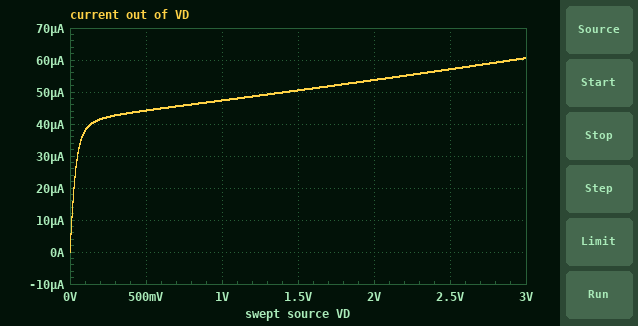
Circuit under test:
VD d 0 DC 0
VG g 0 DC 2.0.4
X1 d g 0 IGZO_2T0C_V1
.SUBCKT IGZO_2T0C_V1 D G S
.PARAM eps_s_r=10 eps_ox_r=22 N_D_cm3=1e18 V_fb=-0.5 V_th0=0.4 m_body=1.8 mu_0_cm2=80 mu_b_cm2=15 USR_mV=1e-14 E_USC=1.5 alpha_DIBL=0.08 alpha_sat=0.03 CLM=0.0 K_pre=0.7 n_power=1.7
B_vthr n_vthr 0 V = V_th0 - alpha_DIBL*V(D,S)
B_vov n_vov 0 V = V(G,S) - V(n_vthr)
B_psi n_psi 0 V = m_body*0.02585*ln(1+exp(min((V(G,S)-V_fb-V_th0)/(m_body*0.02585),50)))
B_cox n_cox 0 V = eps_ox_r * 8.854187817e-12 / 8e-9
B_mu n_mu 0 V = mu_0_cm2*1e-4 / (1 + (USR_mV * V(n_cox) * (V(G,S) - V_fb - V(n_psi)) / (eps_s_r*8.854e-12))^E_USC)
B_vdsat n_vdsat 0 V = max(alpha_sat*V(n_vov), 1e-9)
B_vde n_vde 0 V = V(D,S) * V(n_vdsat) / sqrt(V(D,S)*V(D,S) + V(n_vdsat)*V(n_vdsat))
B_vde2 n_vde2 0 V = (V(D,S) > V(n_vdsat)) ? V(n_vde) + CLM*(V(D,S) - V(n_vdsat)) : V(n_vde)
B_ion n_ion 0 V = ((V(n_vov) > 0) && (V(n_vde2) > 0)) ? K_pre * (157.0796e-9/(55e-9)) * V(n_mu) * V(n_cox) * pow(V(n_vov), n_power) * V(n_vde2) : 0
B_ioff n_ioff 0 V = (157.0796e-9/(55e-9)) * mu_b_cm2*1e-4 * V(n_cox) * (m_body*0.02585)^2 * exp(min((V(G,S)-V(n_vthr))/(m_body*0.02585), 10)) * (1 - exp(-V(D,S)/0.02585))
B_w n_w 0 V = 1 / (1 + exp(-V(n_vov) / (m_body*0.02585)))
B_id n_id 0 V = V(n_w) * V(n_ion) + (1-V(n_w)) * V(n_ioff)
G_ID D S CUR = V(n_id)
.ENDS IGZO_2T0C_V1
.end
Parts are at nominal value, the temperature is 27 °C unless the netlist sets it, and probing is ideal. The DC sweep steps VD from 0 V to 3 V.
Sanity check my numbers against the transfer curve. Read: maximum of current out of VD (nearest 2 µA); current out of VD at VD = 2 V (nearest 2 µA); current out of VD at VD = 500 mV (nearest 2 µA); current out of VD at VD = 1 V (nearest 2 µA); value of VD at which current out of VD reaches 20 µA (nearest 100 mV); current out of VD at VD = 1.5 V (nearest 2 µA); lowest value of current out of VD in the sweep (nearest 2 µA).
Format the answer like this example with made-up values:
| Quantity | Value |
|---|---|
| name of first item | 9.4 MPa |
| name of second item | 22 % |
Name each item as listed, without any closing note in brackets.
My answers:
| Quantity | Value |
|---|---|
| maximum of current out of VD | 60 µA |
| current out of VD at VD = 2 V | 54 µA |
| current out of VD at VD = 500 mV | 44 µA |
| current out of VD at VD = 1 V | 48 µA |
| value of VD at which current out of VD reaches 20 µA | 0 V |
| current out of VD at VD = 1.5 V | 50 µA |
| lowest value of current out of VD in the sweep | 0 A |
